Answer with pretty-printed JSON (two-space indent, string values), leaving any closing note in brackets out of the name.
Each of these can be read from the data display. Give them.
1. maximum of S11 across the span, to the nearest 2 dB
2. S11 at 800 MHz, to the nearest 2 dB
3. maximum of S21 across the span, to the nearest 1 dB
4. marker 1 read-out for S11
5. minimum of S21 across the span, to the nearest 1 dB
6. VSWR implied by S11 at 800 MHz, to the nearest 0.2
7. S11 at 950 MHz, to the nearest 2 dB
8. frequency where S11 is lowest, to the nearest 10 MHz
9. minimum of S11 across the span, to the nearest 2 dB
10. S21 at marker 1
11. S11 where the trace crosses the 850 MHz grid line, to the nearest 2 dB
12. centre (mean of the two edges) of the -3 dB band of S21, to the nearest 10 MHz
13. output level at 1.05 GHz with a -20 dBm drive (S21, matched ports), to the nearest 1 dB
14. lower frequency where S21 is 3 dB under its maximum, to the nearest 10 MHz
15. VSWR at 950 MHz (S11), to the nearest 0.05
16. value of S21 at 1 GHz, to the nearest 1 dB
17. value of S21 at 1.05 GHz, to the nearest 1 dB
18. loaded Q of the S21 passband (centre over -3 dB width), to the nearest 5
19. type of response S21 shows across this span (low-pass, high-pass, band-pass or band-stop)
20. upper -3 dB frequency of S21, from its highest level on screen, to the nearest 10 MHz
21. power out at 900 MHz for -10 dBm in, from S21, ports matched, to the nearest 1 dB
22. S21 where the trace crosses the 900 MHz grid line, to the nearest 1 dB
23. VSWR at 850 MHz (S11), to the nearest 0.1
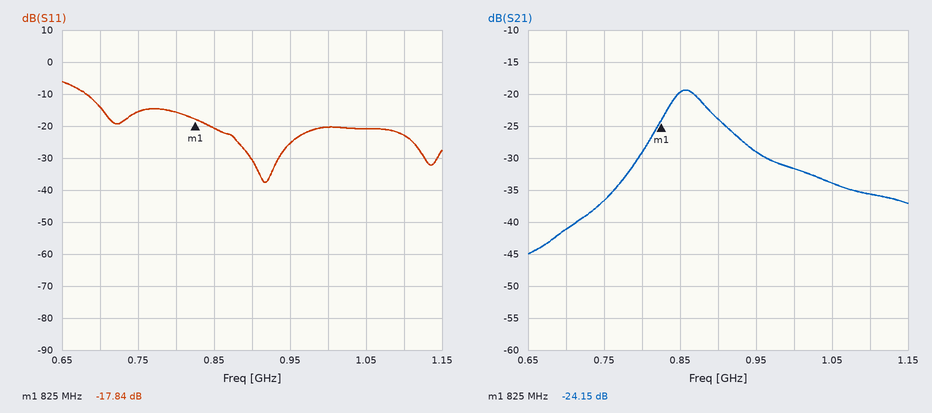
{
  "maximum of S11 across the span, to the nearest 2 dB": "-6 dB",
  "S11 at 800 MHz, to the nearest 2 dB": "-16 dB",
  "maximum of S21 across the span, to the nearest 1 dB": "-19 dB",
  "marker 1 read-out for S11": "-17.84 dB",
  "minimum of S21 across the span, to the nearest 1 dB": "-45 dB",
  "VSWR implied by S11 at 800 MHz, to the nearest 0.2": "1.4",
  "S11 at 950 MHz, to the nearest 2 dB": "-26 dB",
  "frequency where S11 is lowest, to the nearest 10 MHz": "920 MHz",
  "minimum of S11 across the span, to the nearest 2 dB": "-38 dB",
  "S21 at marker 1": "-24.15 dB",
  "S11 where the trace crosses the 850 MHz grid line, to the nearest 2 dB": "-20 dB",
  "centre (mean of the two edges) of the -3 dB band of S21, to the nearest 10 MHz": "860 MHz",
  "output level at 1.05 GHz with a -20 dBm drive (S21, matched ports), to the nearest 1 dB": "-54 dBm",
  "lower frequency where S21 is 3 dB under its maximum, to the nearest 10 MHz": "830 MHz",
  "VSWR at 950 MHz (S11), to the nearest 0.05": "1.10",
  "value of S21 at 1 GHz, to the nearest 1 dB": "-32 dB",
  "value of S21 at 1.05 GHz, to the nearest 1 dB": "-34 dB",
  "loaded Q of the S21 passband (centre over -3 dB width), to the nearest 5": "15",
  "type of response S21 shows across this span": "band-pass",
  "upper -3 dB frequency of S21, from its highest level on screen, to the nearest 10 MHz": "890 MHz",
  "power out at 900 MHz for -10 dBm in, from S21, ports matched, to the nearest 1 dB": "-34 dBm",
  "S21 where the trace crosses the 900 MHz grid line, to the nearest 1 dB": "-24 dB",
  "VSWR at 850 MHz (S11), to the nearest 0.1": "1.2"
}
